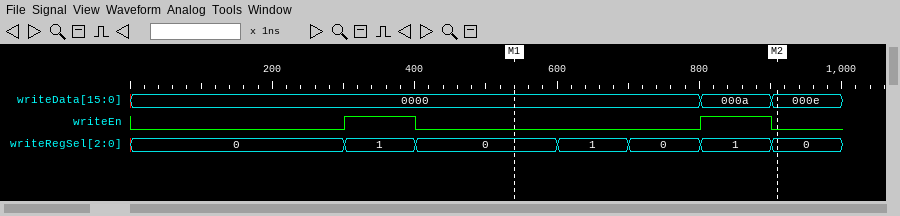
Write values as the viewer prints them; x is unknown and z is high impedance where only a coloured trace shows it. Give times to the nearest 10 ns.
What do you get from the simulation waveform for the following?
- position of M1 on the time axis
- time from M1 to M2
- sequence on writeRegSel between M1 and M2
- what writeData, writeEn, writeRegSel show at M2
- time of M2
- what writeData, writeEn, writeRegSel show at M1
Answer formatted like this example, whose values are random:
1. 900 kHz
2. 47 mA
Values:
1. 540 ns
2. 370 ns
3. 0, 1, 0, 1, 0
4. writeData=000e, writeEn=0, writeRegSel=0
5. 910 ns
6. writeData=0000, writeEn=0, writeRegSel=0
